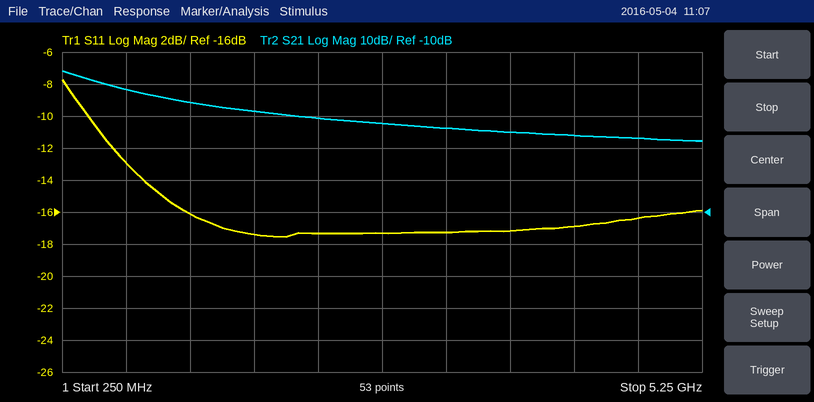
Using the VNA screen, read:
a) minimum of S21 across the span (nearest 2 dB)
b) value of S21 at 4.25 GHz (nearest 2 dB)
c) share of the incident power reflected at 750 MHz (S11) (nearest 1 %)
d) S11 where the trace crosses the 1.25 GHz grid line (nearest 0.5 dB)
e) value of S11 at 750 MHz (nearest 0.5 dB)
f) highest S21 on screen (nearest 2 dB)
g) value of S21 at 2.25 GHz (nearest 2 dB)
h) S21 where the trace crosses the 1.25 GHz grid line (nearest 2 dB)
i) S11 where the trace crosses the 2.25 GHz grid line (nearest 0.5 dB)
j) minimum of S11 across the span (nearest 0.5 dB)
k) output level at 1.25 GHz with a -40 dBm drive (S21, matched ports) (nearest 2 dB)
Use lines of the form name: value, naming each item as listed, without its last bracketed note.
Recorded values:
minimum of S21 across the span: 12 dB
value of S21 at 4.25 GHz: 14 dB
share of the incident power reflected at 750 MHz (S11): 5 %
S11 where the trace crosses the 1.25 GHz grid line: -16.0 dB
value of S11 at 750 MHz: -13.0 dB
highest S21 on screen: 34 dB
value of S21 at 2.25 GHz: 20 dB
S21 where the trace crosses the 1.25 GHz grid line: 24 dB
S11 where the trace crosses the 2.25 GHz grid line: -17.5 dB
minimum of S11 across the span: -17.5 dB
output level at 1.25 GHz with a -40 dBm drive (S21, matched ports): -16 dBm
